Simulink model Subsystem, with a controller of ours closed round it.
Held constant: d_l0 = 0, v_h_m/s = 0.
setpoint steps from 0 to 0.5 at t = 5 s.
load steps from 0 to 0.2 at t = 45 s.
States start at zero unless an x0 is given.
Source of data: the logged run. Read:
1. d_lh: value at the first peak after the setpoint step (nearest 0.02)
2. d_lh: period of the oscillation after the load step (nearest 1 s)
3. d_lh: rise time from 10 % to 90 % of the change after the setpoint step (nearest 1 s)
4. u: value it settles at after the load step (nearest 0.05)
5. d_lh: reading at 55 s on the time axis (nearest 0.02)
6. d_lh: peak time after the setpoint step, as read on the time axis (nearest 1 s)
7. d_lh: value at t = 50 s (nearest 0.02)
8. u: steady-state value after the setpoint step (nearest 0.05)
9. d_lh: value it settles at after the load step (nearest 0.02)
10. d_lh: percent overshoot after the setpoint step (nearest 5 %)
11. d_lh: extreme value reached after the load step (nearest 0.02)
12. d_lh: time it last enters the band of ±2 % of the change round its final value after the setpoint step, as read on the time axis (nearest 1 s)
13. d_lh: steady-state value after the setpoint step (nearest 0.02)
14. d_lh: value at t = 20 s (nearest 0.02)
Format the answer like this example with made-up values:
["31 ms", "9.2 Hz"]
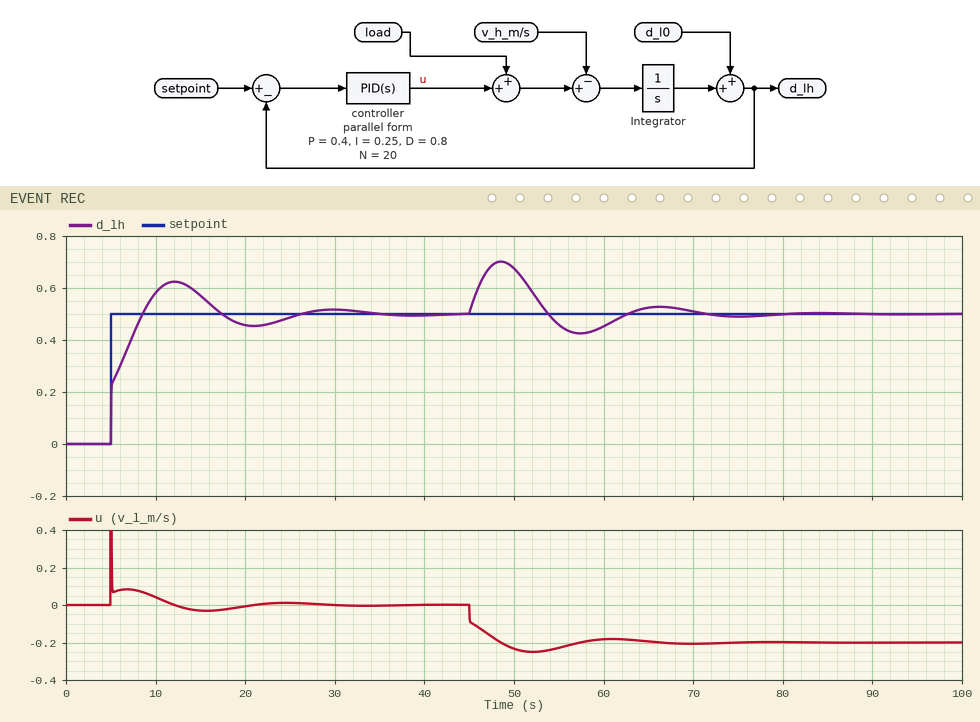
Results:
["0.62", "18 s", "3 s", "-0.20", "0.46", "12 s", "0.68", "0.00", "0.50", "25 %", "0.70", "33 s", "0.50", "0.46"]
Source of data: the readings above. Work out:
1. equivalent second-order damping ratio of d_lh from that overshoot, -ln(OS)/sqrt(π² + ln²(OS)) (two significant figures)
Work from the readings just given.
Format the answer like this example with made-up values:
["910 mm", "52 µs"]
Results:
["0.40"]
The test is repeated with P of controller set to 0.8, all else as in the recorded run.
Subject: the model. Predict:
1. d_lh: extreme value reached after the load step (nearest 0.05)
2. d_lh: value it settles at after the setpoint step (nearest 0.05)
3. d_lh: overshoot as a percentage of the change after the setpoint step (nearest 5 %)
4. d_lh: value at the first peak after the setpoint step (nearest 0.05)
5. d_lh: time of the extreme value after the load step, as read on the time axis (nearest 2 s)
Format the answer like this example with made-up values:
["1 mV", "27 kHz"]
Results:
["0.65", "0.50", "15 %", "0.55", "48 s"]
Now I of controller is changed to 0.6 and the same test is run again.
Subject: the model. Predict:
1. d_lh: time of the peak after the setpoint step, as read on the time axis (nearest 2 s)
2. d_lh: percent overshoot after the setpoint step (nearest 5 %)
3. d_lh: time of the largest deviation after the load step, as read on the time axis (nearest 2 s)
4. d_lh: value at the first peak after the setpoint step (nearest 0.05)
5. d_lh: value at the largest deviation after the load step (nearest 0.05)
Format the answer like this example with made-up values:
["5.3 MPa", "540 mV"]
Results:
["10 s", "30 %", "48 s", "0.65", "0.65"]
